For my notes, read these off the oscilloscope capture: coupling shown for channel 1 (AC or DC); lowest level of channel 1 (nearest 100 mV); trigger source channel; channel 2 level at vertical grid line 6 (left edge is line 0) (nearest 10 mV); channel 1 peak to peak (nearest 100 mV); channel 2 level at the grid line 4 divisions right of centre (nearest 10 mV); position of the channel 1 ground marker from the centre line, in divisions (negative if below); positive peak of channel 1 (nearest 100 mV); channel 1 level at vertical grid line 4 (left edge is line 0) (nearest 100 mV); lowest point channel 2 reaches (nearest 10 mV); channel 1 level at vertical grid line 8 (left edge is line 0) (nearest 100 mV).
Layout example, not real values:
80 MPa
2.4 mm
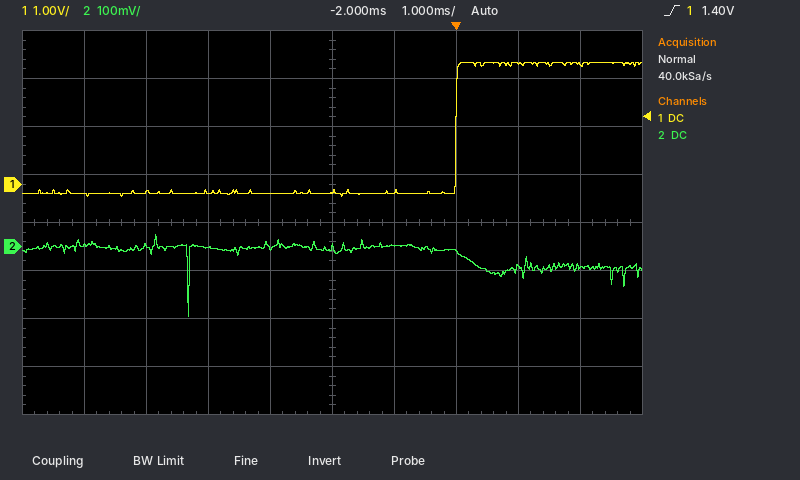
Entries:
DC
-300 mV
channel 1
0 mV
2.8 V
-40 mV
+0.8 div
2.5 V
-200 mV
-150 mV
2.5 V
